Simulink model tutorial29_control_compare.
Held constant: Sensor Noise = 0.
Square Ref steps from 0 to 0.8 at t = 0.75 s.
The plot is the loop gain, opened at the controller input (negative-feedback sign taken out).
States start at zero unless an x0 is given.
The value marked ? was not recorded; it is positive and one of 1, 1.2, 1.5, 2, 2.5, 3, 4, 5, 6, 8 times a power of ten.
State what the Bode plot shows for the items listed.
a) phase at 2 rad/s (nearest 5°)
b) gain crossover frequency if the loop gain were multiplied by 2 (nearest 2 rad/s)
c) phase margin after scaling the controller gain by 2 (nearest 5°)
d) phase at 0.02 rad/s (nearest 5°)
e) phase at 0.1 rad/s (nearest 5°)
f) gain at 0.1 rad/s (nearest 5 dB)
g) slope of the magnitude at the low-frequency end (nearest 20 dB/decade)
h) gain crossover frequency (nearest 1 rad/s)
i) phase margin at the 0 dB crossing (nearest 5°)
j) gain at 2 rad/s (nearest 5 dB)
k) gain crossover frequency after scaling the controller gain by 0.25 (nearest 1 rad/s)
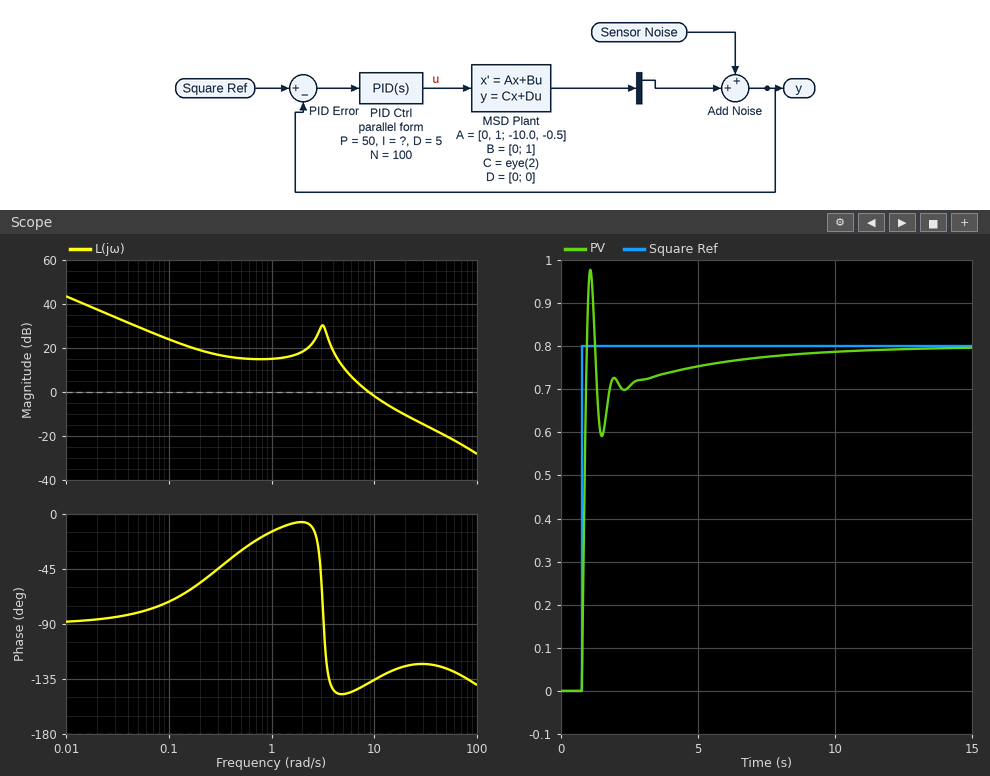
-5°
14 rad/s
50°
-85°
-70°
25 dB
-20 dB/decade
9 rad/s
40°
20 dB
5 rad/s
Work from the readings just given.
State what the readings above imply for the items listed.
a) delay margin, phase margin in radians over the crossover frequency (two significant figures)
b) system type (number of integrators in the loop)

0.078 s
1
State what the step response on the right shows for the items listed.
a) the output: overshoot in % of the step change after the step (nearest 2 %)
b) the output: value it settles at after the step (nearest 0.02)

22 %
0.80
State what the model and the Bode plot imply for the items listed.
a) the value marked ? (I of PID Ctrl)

15
